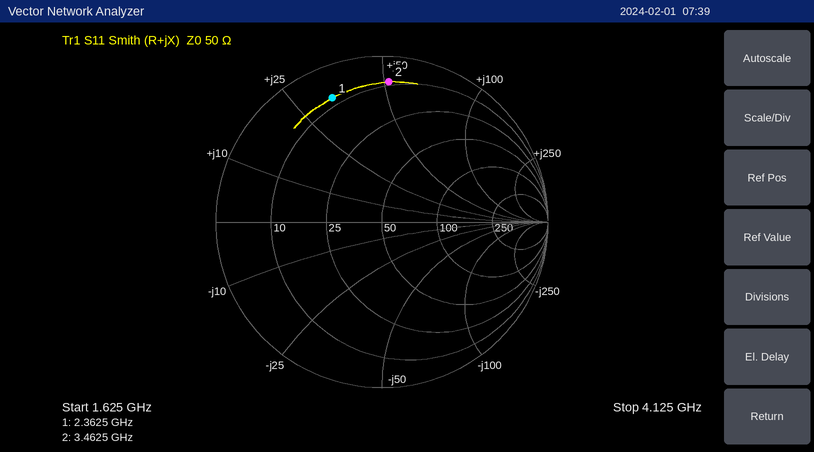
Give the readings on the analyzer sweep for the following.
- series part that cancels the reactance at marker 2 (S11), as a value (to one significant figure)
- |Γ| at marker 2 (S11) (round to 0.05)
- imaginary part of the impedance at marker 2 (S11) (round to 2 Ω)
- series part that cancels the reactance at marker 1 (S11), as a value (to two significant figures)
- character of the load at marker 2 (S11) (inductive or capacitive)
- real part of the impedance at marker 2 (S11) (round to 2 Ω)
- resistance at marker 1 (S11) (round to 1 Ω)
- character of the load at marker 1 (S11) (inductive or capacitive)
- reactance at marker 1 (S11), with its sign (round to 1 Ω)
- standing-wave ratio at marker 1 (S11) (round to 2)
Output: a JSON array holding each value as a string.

["900 fF", "0.85", "+52 Ω", "2.0 pF", "inductive", "8 Ω", "8 Ω", "inductive", "+33 Ω", "10"]
